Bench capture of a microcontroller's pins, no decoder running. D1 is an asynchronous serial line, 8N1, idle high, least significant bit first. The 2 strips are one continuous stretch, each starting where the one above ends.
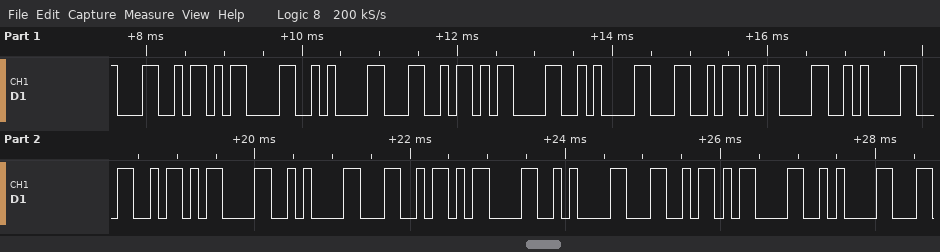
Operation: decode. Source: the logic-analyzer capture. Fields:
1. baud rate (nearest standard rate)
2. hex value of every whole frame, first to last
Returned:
9600 baud
0x4C 0x0D 0x0A 0x4C 0x0D 0x0A 0x4C 0x0D 0x0A 0x4C 0x0D 0x0A 0x4C 0x0D 0x0A 0x4C 0x0D 0x0A
